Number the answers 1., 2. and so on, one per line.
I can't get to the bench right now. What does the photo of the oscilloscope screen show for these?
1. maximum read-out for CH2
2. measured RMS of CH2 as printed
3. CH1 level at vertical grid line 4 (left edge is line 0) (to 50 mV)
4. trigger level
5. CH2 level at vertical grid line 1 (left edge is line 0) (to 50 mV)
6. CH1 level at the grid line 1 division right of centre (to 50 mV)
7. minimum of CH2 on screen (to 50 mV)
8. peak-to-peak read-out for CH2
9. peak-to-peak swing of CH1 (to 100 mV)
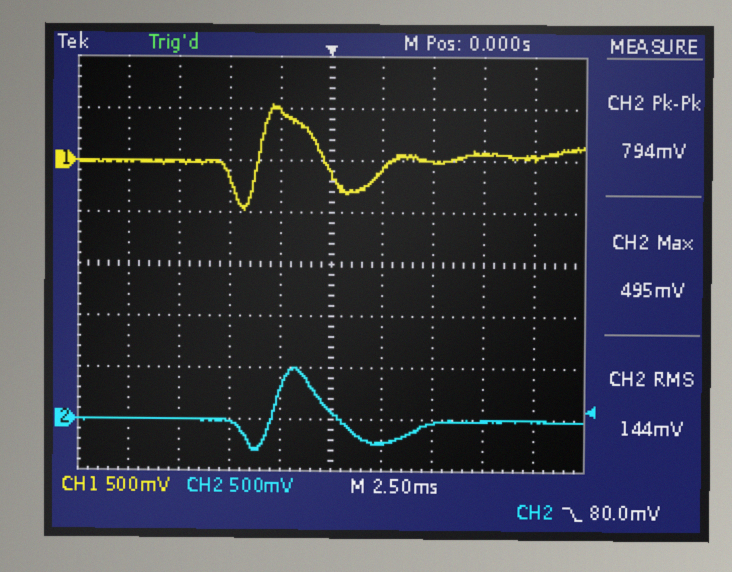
1. 495 mV
2. 144 mV
3. 500 mV
4. 80.0 mV
5. 0 mV
6. -100 mV
7. -300 mV
8. 794 mV
9. 1.00 V
